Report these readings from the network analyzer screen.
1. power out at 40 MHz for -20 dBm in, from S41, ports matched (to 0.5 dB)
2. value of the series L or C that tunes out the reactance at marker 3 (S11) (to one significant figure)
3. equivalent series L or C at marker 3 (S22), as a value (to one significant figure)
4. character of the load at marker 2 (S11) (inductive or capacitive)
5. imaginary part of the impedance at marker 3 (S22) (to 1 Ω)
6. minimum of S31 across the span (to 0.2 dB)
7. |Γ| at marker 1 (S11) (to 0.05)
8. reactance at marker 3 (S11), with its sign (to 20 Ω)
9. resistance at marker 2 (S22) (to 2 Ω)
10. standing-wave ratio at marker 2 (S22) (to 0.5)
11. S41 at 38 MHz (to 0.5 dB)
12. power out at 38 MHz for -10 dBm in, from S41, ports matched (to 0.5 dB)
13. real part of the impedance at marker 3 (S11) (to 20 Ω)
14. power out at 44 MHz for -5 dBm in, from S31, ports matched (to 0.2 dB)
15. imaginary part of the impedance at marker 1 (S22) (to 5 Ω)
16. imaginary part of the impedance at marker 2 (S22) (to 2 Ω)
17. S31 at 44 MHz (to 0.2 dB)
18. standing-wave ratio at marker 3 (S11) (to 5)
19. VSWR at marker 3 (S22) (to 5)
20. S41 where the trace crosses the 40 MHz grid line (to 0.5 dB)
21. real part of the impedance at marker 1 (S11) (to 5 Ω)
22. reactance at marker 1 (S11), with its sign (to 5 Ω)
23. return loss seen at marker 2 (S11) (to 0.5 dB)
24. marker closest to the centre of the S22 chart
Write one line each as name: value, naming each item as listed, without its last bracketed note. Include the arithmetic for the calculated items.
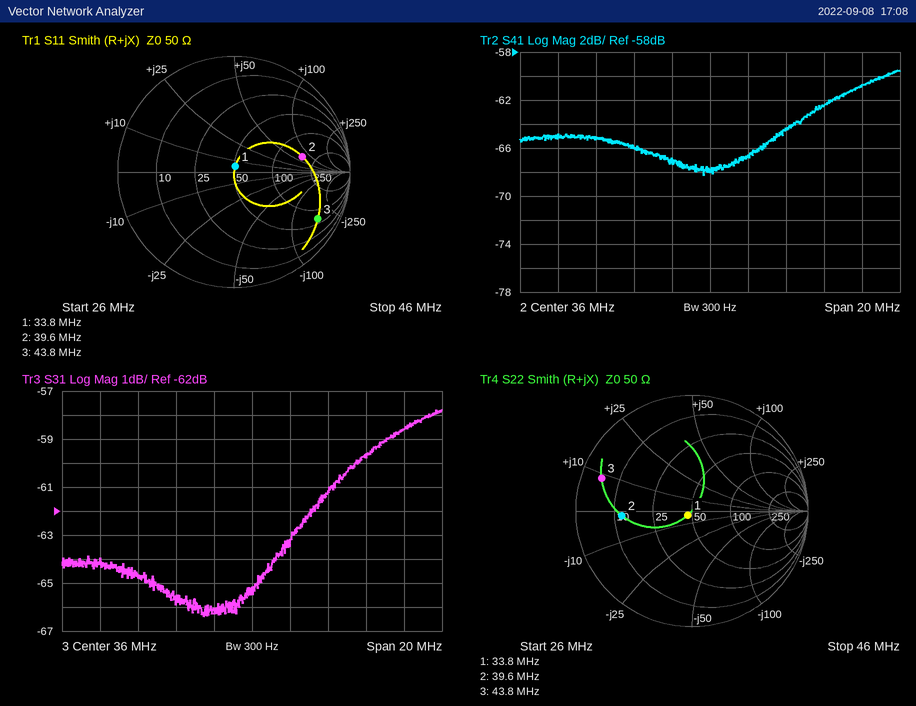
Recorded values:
power out at 40 MHz for -20 dBm in, from S41, ports matched: -20 dBm + (-64.5 dB) = -84.5 dBm
value of the series L or C that tunes out the reactance at marker 3 (S11): L = 160 Ω/(2π × 43.8 MHz) ≈ 581 nH, so 600 nH to one significant figure
equivalent series L or C at marker 3 (S22), as a value: L = 9 Ω/(2π × 43.8 MHz) ≈ 32.7 nH, so 30 nH to one significant figure
character of the load at marker 2 (S11): inductive
imaginary part of the impedance at marker 3 (S22): +9 Ω
minimum of S31 across the span: -66.4 dB
|Γ| at marker 1 (S11): 0.05
reactance at marker 3 (S11), with its sign: -160 Ω
resistance at marker 2 (S22): 12 Ω
standing-wave ratio at marker 2 (S22): 4.0
S41 at 38 MHz: -66.5 dB
power out at 38 MHz for -10 dBm in, from S41, ports matched: -10 dBm + (-66.5 dB) = -76.5 dBm
real part of the impedance at marker 3 (S11): 60 Ω
power out at 44 MHz for -5 dBm in, from S31, ports matched: -5 dBm + (-58.6 dB) = -63.6 dBm
imaginary part of the impedance at marker 1 (S22): -5 Ω
imaginary part of the impedance at marker 2 (S22): -2 Ω
S31 at 44 MHz: -58.6 dB
standing-wave ratio at marker 3 (S11): 10
VSWR at marker 3 (S22): 10
S41 where the trace crosses the 40 MHz grid line: -64.5 dB
real part of the impedance at marker 1 (S11): 50 Ω
reactance at marker 1 (S11), with its sign: +5 Ω
return loss seen at marker 2 (S11): 4.5 dB
marker closest to the centre of the S22 chart: marker 1
